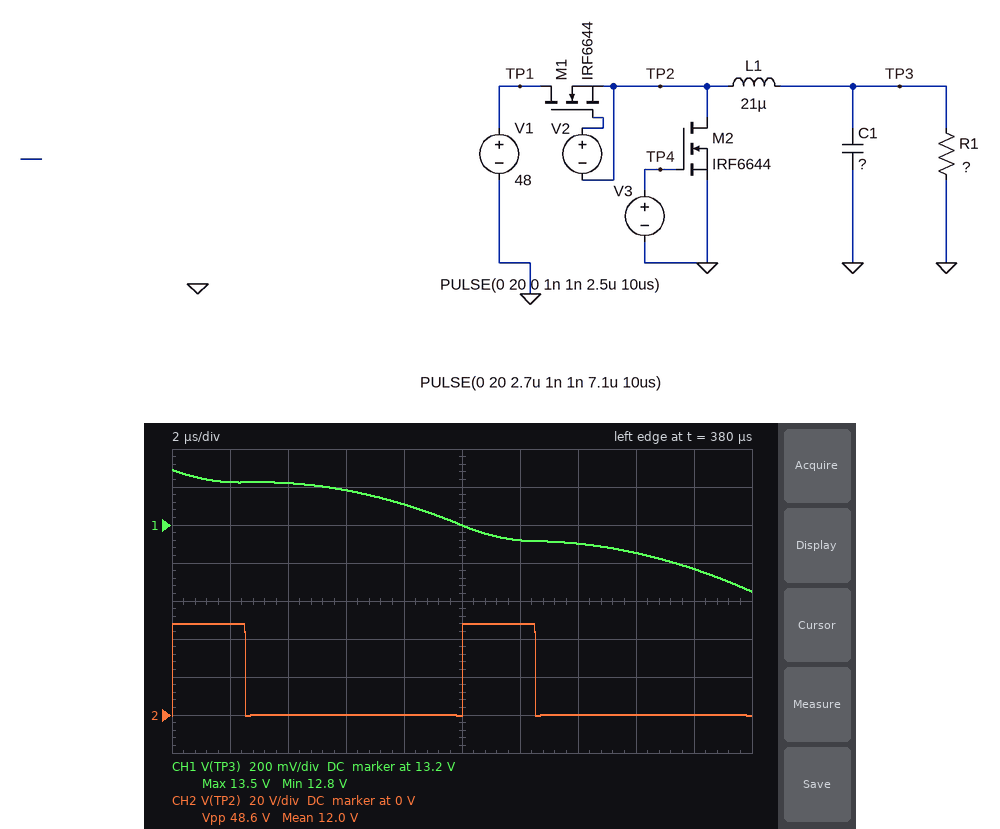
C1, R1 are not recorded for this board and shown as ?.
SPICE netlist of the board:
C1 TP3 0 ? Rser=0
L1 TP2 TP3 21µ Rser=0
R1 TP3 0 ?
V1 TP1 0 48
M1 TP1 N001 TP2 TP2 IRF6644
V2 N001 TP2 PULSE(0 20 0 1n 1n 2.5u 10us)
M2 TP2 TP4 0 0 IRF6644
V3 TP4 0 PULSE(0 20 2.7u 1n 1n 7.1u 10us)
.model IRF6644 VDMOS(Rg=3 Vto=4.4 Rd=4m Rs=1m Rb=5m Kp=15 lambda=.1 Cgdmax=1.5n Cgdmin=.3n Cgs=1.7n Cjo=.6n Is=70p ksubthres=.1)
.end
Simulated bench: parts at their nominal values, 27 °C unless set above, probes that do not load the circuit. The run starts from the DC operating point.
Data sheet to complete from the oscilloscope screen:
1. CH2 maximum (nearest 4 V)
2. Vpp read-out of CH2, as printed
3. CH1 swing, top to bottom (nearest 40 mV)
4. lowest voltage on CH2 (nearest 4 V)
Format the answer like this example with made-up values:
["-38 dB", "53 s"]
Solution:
["48 V", "48.6 V", "640 mV", "0 V"]
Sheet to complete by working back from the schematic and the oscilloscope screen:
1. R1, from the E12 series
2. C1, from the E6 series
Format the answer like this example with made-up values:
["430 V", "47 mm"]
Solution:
["1.8 Ω", "68 µF"]
